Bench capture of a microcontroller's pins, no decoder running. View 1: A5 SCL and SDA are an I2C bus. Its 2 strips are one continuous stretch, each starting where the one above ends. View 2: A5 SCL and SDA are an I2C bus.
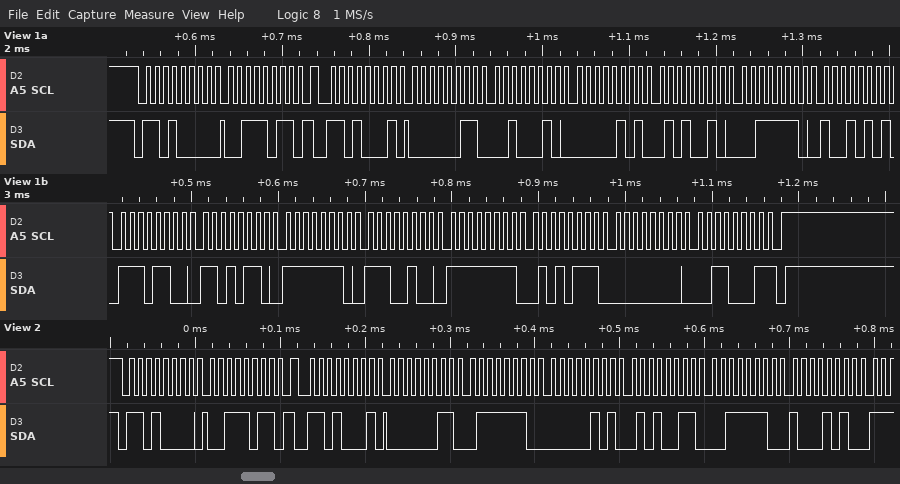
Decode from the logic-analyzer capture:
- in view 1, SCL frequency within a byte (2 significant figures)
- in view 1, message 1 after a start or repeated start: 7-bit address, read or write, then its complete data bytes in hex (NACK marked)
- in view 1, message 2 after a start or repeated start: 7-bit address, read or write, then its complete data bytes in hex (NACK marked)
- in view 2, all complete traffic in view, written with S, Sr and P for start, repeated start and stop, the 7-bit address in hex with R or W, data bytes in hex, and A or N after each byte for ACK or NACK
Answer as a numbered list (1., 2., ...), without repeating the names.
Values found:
1. 100 kHz
2. 0x68 write: 3B
3. 0x68 read: 03 22 05 52 3E 95 EC D6 FE E4 FF 57 00 31 NACK
4. S 68W A 3B A Sr 68R A 03 A 7E A 05 A 53 A 3E A 8A A
